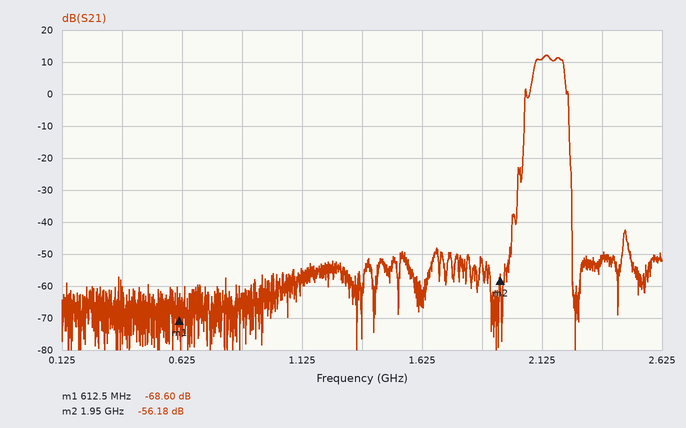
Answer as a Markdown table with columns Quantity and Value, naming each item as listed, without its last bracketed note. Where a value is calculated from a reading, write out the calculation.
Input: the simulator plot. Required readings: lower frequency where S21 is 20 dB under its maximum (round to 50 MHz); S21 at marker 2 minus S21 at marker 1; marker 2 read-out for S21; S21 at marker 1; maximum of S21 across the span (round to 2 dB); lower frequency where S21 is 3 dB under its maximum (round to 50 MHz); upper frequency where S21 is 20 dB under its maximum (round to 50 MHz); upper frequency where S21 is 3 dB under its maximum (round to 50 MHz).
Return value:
| Quantity | Value |
|---|---|
| lower frequency where S21 is 20 dB under its maximum | 2.05 GHz |
| S21 at marker 2 minus S21 at marker 1 | -56.18 − (-68.6) = 12.42 dB |
| marker 2 read-out for S21 | -56.18 dB |
| S21 at marker 1 | -68.60 dB |
| maximum of S21 across the span | 12 dB |
| lower frequency where S21 is 3 dB under its maximum | 2.10 GHz |
| upper frequency where S21 is 20 dB under its maximum | 2.25 GHz |
| upper frequency where S21 is 3 dB under its maximum | 2.20 GHz |
